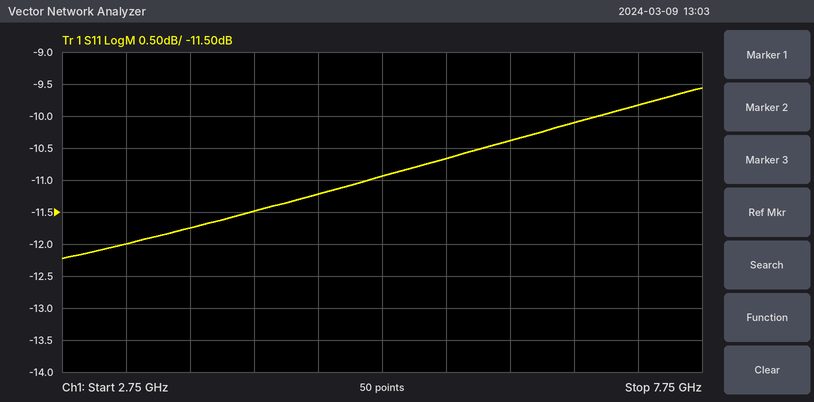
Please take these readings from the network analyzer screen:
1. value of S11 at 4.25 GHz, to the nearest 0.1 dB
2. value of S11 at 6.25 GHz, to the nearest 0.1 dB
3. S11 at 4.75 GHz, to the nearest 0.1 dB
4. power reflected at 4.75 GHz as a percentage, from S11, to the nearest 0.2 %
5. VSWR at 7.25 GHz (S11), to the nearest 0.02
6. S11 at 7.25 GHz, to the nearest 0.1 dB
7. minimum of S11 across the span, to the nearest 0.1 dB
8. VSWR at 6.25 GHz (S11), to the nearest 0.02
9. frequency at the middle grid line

-11.5 dB
-10.4 dB
-11.2 dB
7.6 %
1.96
-9.8 dB
-12.2 dB
1.86
5.25 GHz
